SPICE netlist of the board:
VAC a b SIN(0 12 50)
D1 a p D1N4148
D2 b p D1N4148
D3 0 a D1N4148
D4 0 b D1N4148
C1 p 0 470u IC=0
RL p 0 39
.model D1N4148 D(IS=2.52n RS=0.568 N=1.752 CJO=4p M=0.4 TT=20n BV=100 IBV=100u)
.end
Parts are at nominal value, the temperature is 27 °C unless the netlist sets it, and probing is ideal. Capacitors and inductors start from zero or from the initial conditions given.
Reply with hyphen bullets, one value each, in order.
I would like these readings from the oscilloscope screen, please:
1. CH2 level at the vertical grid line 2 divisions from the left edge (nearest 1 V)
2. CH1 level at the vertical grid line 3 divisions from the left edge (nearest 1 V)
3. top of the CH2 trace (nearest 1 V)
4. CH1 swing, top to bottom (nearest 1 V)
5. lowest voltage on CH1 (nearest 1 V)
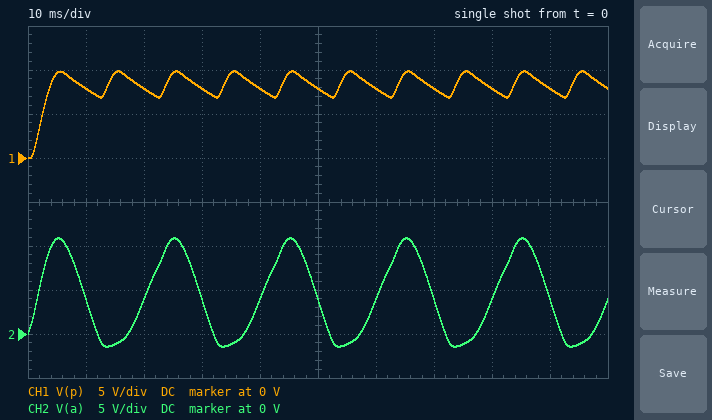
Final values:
- 4 V
- 8 V
- 11 V
- 10 V
- 0 V
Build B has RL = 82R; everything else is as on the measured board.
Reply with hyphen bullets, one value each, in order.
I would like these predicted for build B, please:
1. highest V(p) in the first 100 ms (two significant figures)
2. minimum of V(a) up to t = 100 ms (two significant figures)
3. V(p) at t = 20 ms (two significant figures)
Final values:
- 10 V
- -1.2 V
- 9.0 V
